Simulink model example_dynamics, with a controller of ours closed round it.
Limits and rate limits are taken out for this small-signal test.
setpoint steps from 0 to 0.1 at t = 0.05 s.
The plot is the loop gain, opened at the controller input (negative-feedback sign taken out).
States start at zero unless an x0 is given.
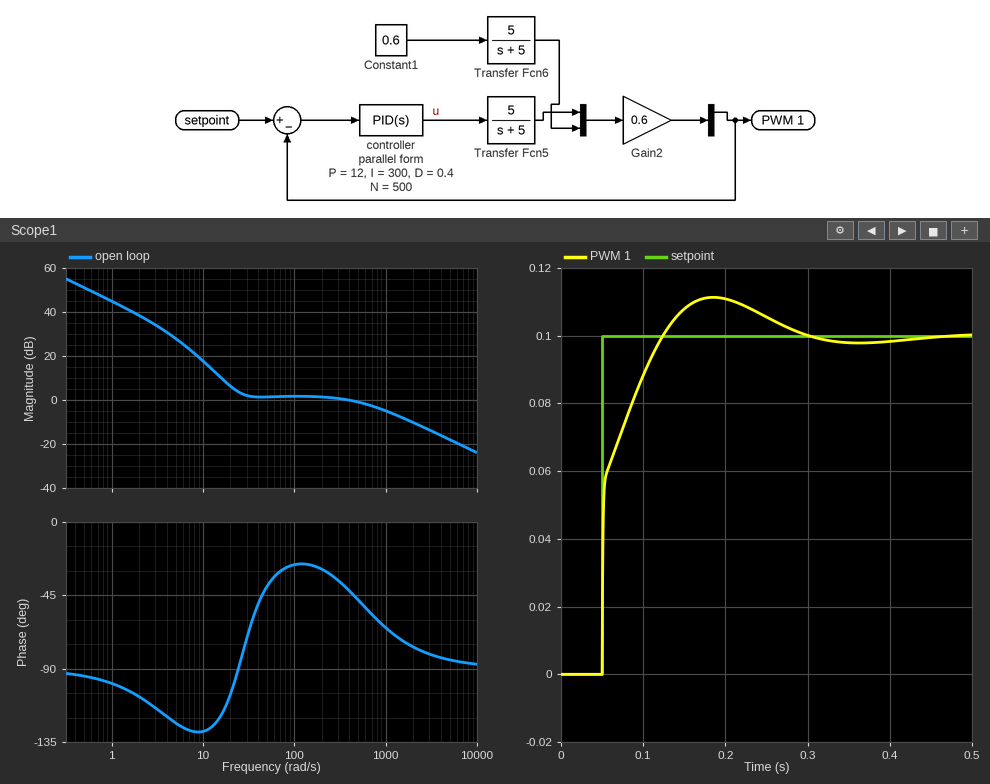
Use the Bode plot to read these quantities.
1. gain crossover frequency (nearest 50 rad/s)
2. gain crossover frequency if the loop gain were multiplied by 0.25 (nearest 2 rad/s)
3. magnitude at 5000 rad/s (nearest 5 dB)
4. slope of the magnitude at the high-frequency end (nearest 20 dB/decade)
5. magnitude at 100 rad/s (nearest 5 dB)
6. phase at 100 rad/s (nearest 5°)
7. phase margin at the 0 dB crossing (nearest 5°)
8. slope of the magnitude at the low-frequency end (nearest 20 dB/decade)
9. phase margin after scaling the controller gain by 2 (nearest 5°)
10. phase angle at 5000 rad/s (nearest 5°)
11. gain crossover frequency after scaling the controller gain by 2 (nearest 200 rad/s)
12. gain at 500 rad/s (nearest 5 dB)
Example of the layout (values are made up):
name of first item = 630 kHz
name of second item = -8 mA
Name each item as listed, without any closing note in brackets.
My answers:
gain crossover frequency = 400 rad/s
gain crossover frequency if the loop gain were multiplied by 0.25 = 14 rad/s
magnitude at 5000 rad/s = -20 dB
slope of the magnitude at the high-frequency end = -20 dB/decade
magnitude at 100 rad/s = 0 dB
phase at 100 rad/s = -25°
phase margin at the 0 dB crossing = 140°
slope of the magnitude at the low-frequency end = -20 dB/decade
phase margin after scaling the controller gain by 2 = 110°
phase angle at 5000 rad/s = -85°
gain crossover frequency after scaling the controller gain by 2 = 1200 rad/s
gain at 500 rad/s = 0 dB
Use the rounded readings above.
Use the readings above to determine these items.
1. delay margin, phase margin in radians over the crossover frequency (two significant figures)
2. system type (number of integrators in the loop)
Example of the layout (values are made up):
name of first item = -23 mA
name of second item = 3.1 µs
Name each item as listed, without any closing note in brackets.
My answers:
delay margin, phase margin in radians over the crossover frequency = 0.0061 s
system type = 1
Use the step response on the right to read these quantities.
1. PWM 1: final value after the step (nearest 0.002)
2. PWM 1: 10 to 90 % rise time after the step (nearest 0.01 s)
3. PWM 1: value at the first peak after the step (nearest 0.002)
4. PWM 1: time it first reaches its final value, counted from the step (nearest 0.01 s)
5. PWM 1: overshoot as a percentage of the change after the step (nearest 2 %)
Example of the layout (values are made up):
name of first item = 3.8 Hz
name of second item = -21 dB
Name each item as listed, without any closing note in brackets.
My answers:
PWM 1: final value after the step = 0.100
PWM 1: 10 to 90 % rise time after the step = 0.05 s
PWM 1: value at the first peak after the step = 0.112
PWM 1: time it first reaches its final value, counted from the step = 0.07 s
PWM 1: overshoot as a percentage of the change after the step = 12 %
